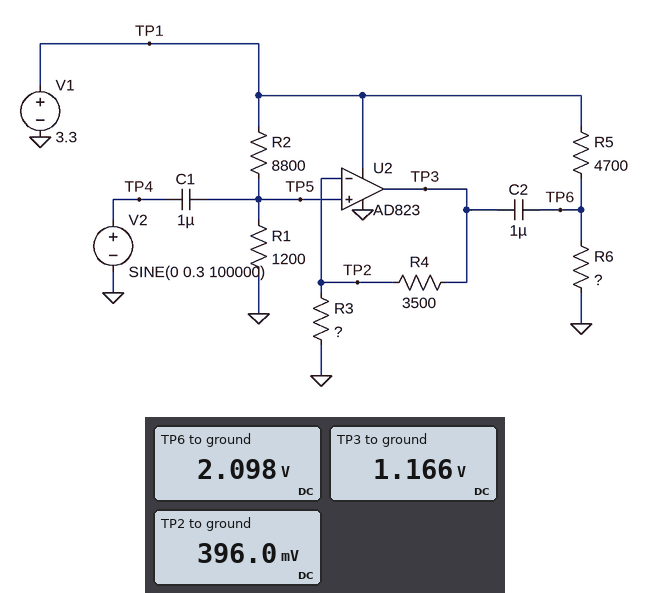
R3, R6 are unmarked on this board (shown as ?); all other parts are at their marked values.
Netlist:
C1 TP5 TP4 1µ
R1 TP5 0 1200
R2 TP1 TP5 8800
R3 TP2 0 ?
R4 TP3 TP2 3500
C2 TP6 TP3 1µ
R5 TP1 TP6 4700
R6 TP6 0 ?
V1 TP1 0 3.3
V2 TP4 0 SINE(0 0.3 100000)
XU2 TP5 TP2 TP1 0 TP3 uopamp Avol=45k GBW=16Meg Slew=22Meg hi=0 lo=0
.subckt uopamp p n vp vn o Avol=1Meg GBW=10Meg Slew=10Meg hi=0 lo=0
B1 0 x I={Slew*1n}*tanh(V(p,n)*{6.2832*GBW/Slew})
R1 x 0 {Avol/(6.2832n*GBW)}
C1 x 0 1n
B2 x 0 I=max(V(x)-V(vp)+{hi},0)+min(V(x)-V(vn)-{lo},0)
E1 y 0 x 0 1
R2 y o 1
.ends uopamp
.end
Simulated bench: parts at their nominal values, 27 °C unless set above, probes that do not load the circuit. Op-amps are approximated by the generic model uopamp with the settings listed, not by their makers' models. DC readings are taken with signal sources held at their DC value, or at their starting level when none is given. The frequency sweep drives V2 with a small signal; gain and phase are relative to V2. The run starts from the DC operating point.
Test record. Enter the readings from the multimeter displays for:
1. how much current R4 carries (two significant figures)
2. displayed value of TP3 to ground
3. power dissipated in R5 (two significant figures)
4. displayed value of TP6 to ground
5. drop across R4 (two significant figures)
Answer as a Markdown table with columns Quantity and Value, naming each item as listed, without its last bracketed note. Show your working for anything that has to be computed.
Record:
| Quantity | Value |
|---|---|
| how much current R4 carries | (1.166 V - 396 mV) / 3.5 kΩ = 220 µA |
| displayed value of TP3 to ground | 1.166 V |
| power dissipated in R5 | (3.3 V - 2.098 V)^2 / 4.7 kΩ = 310 µW |
| displayed value of TP6 to ground | 2.098 V |
| drop across R4 | 1.166 V - 396 mV = 770 mV |
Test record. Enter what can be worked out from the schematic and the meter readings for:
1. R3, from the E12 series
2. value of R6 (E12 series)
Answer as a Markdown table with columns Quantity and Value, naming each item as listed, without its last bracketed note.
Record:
| Quantity | Value |
|---|---|
| R3, from the E12 series | 1.8 kΩ |
| value of R6 | 8.2 kΩ |
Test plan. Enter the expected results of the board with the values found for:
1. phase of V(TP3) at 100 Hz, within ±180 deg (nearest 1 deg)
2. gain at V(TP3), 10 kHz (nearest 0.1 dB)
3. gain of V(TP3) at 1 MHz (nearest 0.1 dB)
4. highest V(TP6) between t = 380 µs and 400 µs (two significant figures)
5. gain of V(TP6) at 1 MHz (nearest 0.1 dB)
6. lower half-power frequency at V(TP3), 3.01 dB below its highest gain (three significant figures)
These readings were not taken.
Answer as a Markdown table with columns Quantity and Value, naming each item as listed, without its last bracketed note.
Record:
| Quantity | Value |
|---|---|
| phase of V(TP3) at 100 Hz, within ±180 deg | 56 deg |
| gain at V(TP3), 10 kHz | 9.4 dB |
| gain of V(TP3) at 1 MHz | 9.2 dB |
| highest V(TP6) between t = 380 µs and 400 µs | 3.0 V |
| gain of V(TP6) at 1 MHz | 9.2 dB |
| lower half-power frequency at V(TP3), 3.01 dB below its highest gain | 151 Hz |
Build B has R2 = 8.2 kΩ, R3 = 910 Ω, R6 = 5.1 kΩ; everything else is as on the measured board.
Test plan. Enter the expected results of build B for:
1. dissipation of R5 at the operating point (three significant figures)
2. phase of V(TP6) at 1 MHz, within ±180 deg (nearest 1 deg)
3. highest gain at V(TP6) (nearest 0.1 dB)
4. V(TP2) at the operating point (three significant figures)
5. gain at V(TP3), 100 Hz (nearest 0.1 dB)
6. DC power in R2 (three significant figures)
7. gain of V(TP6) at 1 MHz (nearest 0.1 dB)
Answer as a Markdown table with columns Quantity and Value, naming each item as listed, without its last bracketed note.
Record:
| Quantity | Value |
|---|---|
| dissipation of R5 at the operating point | 533 µW |
| phase of V(TP6) at 1 MHz, within ±180 deg | -17 deg |
| highest gain at V(TP6) | 13.7 dB |
| V(TP2) at the operating point | 421 mV |
| gain at V(TP3), 100 Hz | 8.5 dB |
| DC power in R2 | 1.01 mW |
| gain of V(TP6) at 1 MHz | 13.3 dB |
